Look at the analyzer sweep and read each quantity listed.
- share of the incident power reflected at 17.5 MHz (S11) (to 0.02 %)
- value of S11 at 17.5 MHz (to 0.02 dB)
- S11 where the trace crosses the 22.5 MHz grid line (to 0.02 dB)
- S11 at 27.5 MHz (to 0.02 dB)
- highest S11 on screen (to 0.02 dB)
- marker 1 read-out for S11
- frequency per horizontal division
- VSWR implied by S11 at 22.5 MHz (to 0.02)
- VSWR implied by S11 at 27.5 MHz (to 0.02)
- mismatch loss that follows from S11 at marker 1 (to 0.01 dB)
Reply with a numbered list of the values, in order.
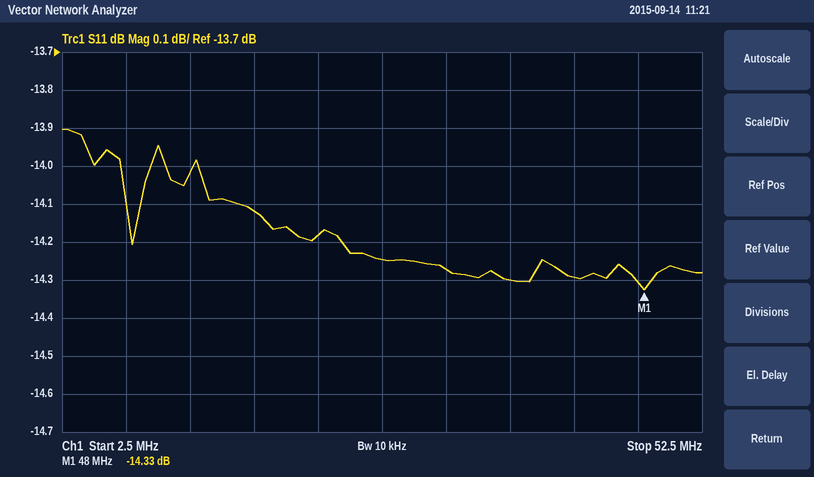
1. 3.88 %
2. -14.12 dB
3. -14.18 dB
4. -14.24 dB
5. -13.90 dB
6. -14.33 dB
7. 5 MHz
8. 1.48
9. 1.48
10. 0.16 dB
